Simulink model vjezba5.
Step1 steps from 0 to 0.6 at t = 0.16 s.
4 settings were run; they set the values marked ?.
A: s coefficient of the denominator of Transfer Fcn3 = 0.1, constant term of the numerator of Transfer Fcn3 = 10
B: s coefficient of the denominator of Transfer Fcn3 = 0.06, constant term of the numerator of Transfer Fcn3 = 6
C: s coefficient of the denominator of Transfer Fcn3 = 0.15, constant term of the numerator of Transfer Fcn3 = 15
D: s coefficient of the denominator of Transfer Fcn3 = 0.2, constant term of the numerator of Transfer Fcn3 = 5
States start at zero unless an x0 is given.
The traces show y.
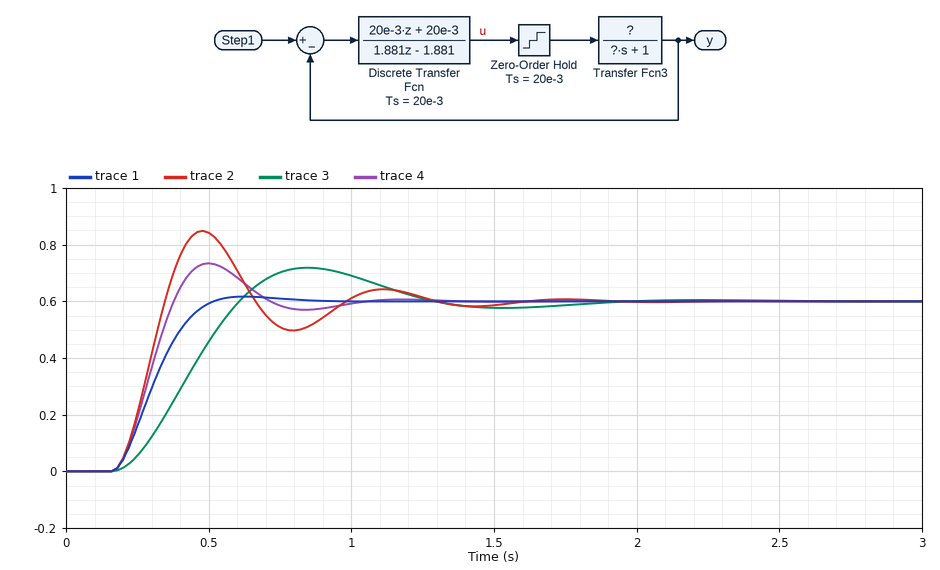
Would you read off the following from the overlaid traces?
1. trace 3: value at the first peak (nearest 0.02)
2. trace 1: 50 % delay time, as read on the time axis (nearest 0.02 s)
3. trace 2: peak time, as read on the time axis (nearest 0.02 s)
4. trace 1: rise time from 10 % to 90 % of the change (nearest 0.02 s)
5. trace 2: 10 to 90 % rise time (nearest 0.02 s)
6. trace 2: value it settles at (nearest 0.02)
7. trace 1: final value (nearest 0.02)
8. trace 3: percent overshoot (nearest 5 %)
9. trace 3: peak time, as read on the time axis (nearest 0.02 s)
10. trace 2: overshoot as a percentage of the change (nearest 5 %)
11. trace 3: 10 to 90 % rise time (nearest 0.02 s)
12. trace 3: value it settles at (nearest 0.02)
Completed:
0.72
0.30 s
0.48 s
0.22 s
0.12 s
0.60
0.60
20 %
0.84 s
40 %
0.30 s
0.60
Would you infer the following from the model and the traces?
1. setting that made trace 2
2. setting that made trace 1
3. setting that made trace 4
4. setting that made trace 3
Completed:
C
B
A
D
